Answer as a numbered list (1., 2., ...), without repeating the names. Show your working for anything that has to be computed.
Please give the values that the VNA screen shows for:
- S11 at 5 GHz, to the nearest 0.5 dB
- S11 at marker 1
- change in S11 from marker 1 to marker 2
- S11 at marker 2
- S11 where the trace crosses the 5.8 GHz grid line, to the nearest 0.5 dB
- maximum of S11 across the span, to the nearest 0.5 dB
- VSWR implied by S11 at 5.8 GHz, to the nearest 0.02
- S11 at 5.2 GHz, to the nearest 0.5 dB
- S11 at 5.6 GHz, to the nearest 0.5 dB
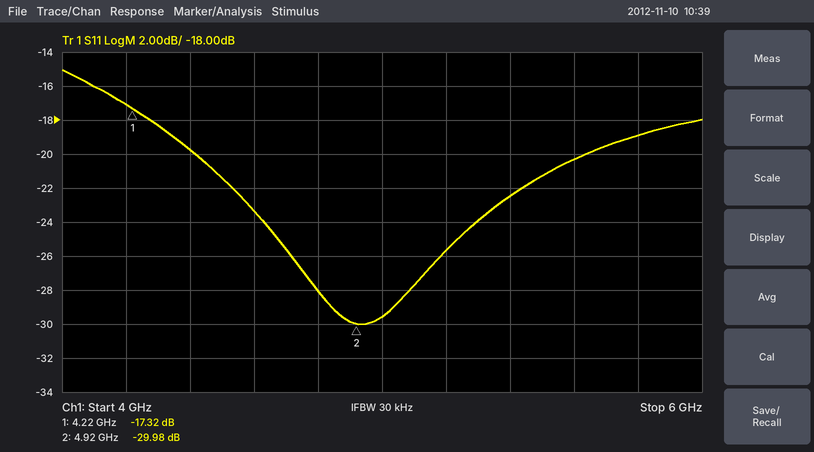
1. -29.5 dB
2. -17.32 dB
3. -29.98 − (-17.32) = -12.66 dB
4. -29.98 dB
5. -19.0 dB
6. -15.0 dB
7. |Γ| = 10^(-19/20) = 0.1122; VSWR = (1 + 0.1122)/(1 − 0.1122) ≈ 1.25, so 1.26 to the nearest 0.02
8. -25.5 dB
9. -20.5 dB
